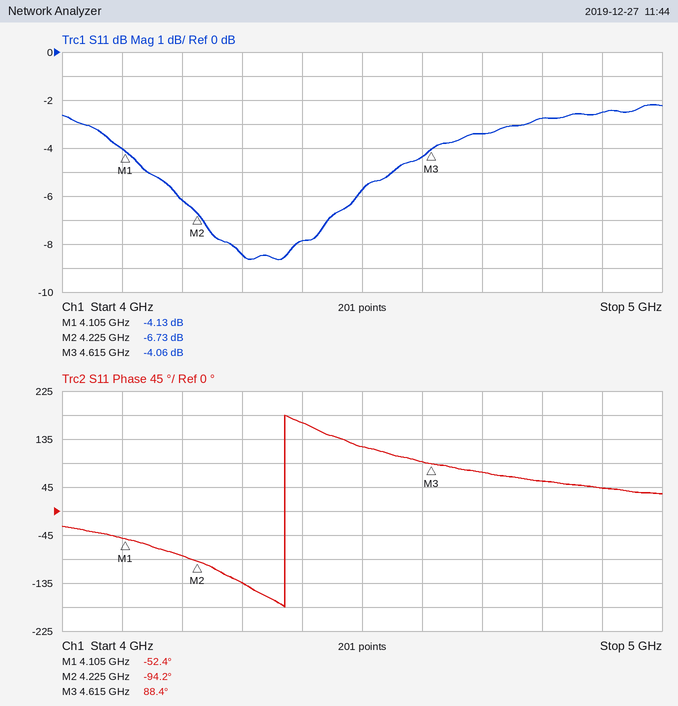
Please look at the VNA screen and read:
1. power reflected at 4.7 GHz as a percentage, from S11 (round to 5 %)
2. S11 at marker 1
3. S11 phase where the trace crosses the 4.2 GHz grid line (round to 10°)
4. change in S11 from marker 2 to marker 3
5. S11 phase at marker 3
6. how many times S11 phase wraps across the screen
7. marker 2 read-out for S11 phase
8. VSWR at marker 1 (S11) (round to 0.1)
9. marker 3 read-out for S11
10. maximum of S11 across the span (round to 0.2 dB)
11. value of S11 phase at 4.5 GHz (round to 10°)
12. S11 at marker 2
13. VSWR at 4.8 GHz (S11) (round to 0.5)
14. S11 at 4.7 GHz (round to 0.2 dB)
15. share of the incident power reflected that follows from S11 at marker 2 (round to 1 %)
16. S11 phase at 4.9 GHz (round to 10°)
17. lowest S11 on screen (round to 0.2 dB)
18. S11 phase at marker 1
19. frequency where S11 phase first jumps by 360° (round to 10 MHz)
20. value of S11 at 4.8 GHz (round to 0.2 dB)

45 %
-4.13 dB
-80°
2.67 dB
88.4°
1
-94.2°
4.3
-4.06 dB
-2.2 dB
120°
-6.73 dB
6.5
-3.4 dB
21 %
40°
-8.6 dB
-52.4°
4.37 GHz
-2.8 dB
